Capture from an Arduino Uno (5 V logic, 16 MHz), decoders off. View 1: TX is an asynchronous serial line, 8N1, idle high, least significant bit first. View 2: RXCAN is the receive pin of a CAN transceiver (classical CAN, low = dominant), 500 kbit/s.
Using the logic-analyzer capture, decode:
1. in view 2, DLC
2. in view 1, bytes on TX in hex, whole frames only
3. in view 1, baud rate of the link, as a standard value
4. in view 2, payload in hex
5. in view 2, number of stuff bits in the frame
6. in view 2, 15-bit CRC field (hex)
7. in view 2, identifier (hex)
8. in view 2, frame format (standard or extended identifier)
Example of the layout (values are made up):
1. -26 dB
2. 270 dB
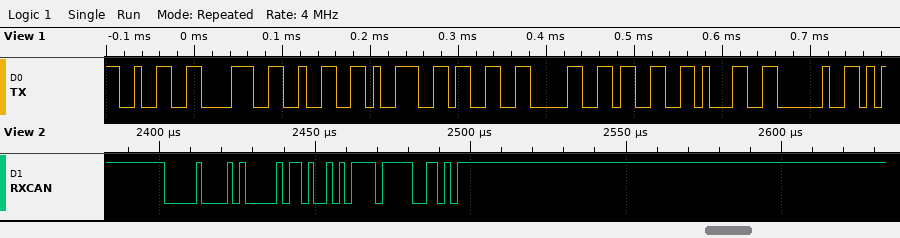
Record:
1. 1
2. 32 38 32 39 33 30 33 31 20
3. 115200 baud
4. A5
5. 3
6. 0x3DF6
7. 0x005
8. standard
